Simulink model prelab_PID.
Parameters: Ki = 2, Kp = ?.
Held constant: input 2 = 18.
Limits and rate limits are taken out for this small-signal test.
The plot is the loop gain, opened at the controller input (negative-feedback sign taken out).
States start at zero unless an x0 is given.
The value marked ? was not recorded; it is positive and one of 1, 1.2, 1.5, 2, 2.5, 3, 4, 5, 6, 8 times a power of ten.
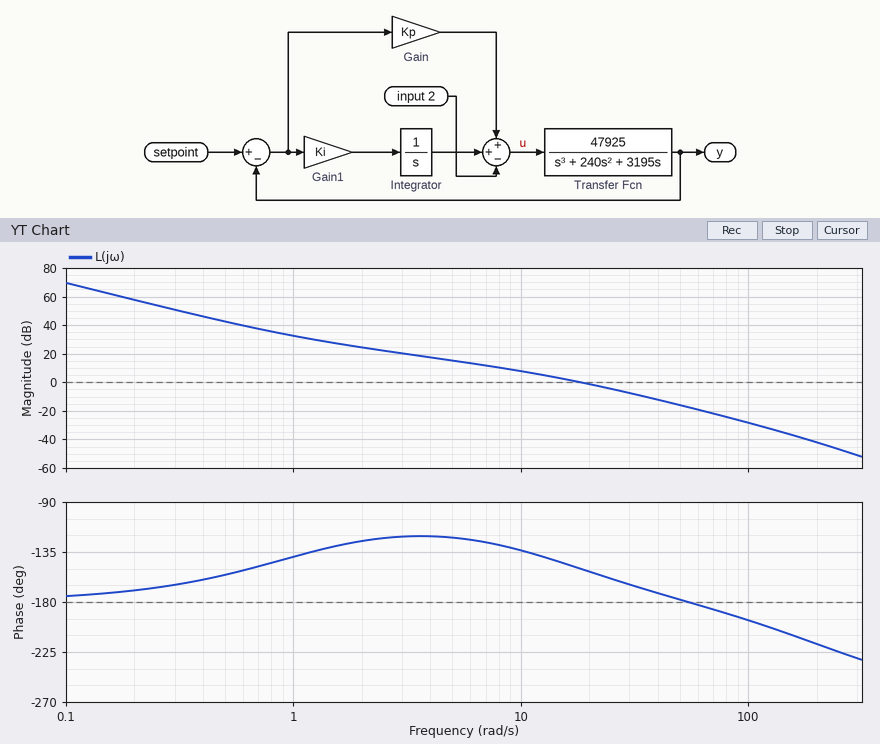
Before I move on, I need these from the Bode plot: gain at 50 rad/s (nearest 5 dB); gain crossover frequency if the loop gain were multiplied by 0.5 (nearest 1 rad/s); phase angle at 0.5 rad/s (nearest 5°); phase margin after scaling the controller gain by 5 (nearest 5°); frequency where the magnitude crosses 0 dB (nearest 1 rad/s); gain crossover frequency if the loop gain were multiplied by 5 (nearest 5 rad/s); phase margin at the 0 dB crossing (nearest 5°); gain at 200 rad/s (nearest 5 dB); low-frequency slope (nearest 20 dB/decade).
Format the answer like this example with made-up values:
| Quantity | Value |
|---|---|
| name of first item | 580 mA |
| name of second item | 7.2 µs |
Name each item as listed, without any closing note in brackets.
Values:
| Quantity | Value |
|---|---|
| gain at 50 rad/s | -15 dB |
| gain crossover frequency if the loop gain were multiplied by 0.5 | 12 rad/s |
| phase angle at 0.5 rad/s | -155° |
| phase margin after scaling the controller gain by 5 | 5° |
| frequency where the magnitude crosses 0 dB | 18 rad/s |
| gain crossover frequency if the loop gain were multiplied by 5 | 45 rad/s |
| phase margin at the 0 dB crossing | 30° |
| gain at 200 rad/s | -40 dB |
| low-frequency slope | -40 dB/decade |
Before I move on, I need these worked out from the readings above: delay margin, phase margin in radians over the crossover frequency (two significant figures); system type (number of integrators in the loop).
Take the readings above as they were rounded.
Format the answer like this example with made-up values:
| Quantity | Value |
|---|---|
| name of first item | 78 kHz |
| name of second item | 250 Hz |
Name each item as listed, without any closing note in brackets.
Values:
| Quantity | Value |
|---|---|
| delay margin, phase margin in radians over the crossover frequency | 0.029 s |
| system type | 2 |
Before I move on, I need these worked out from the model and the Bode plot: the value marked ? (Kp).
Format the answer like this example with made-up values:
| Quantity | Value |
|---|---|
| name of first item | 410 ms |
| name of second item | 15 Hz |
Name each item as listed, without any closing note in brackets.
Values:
| Quantity | Value |
|---|---|
| the value marked ? | 2 |
